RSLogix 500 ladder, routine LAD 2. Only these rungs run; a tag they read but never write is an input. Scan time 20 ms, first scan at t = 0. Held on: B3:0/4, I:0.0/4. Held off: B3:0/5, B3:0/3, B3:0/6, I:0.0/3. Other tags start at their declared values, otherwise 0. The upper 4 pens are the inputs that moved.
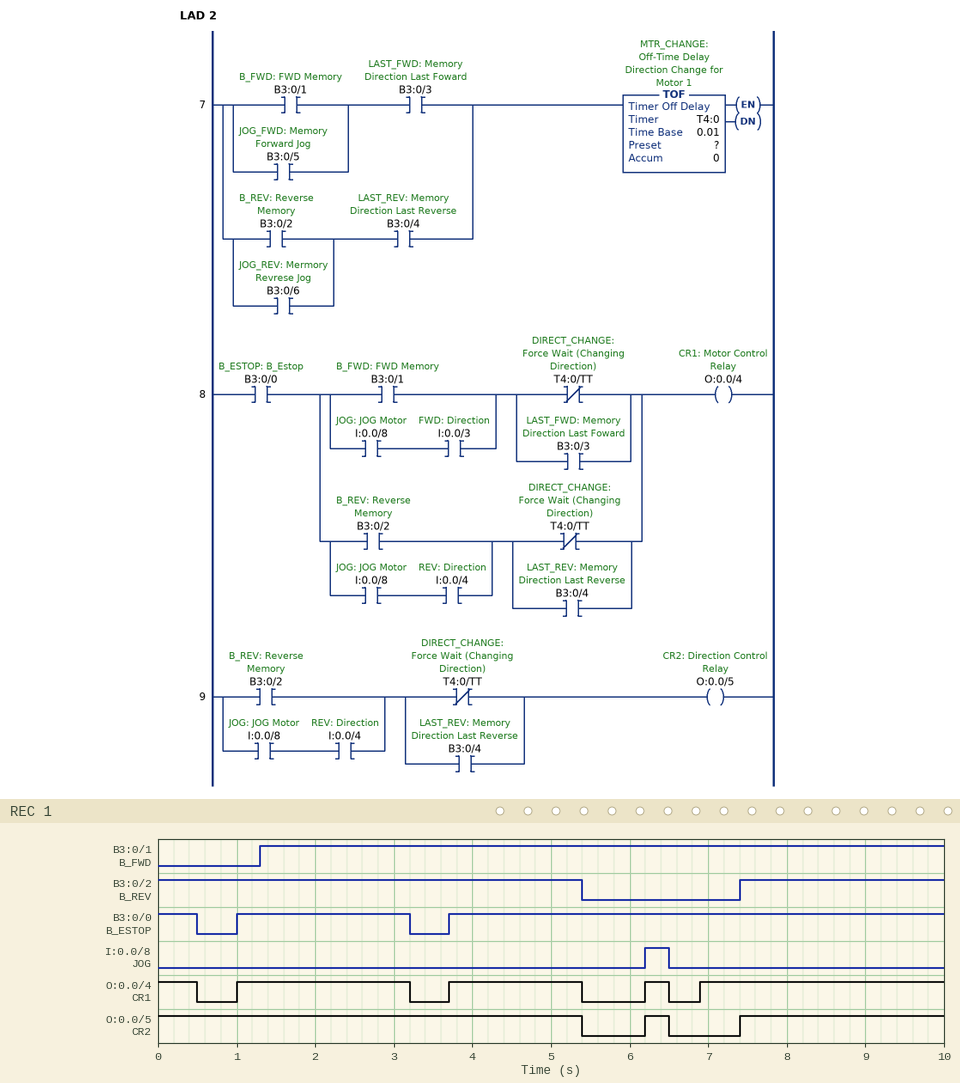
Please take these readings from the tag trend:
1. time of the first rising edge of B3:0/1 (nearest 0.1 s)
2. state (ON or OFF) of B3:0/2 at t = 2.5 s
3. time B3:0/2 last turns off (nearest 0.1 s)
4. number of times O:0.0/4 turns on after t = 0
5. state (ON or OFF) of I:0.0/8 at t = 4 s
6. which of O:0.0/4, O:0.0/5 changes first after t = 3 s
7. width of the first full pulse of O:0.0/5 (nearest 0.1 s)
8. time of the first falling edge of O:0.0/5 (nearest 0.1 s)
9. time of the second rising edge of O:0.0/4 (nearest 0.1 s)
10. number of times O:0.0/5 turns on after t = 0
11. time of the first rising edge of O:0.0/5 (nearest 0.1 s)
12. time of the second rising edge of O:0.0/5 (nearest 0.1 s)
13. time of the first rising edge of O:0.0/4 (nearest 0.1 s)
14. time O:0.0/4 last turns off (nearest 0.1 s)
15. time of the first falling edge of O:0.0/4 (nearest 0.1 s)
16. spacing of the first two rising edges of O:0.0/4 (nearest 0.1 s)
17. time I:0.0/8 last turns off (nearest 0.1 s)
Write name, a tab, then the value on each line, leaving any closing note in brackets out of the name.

time of the first rising edge of B3:0/1	1.3 s
state (ON or OFF) of B3:0/2 at t = 2.5 s	ON
time B3:0/2 last turns off	5.4 s
number of times O:0.0/4 turns on after t = 0	4
state (ON or OFF) of I:0.0/8 at t = 4 s	OFF
which of O:0.0/4, O:0.0/5 changes first after t = 3 s	O:0.0/4
width of the first full pulse of O:0.0/5	0.3 s
time of the first falling edge of O:0.0/5	5.4 s
time of the second rising edge of O:0.0/4	3.7 s
number of times O:0.0/5 turns on after t = 0	2
time of the first rising edge of O:0.0/5	6.2 s
time of the second rising edge of O:0.0/5	7.4 s
time of the first rising edge of O:0.0/4	1.0 s
time O:0.0/4 last turns off	6.5 s
time of the first falling edge of O:0.0/4	0.5 s
spacing of the first two rising edges of O:0.0/4	2.7 s
time I:0.0/8 last turns off	6.5 s
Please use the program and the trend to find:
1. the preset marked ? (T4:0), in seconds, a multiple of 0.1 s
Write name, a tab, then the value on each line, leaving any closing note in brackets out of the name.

the preset marked ? (T4:0), in seconds, a multiple of 0.1 s	1.5 s
